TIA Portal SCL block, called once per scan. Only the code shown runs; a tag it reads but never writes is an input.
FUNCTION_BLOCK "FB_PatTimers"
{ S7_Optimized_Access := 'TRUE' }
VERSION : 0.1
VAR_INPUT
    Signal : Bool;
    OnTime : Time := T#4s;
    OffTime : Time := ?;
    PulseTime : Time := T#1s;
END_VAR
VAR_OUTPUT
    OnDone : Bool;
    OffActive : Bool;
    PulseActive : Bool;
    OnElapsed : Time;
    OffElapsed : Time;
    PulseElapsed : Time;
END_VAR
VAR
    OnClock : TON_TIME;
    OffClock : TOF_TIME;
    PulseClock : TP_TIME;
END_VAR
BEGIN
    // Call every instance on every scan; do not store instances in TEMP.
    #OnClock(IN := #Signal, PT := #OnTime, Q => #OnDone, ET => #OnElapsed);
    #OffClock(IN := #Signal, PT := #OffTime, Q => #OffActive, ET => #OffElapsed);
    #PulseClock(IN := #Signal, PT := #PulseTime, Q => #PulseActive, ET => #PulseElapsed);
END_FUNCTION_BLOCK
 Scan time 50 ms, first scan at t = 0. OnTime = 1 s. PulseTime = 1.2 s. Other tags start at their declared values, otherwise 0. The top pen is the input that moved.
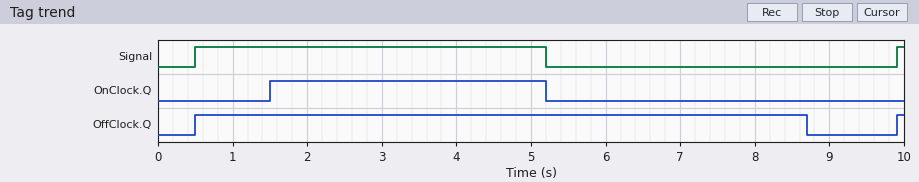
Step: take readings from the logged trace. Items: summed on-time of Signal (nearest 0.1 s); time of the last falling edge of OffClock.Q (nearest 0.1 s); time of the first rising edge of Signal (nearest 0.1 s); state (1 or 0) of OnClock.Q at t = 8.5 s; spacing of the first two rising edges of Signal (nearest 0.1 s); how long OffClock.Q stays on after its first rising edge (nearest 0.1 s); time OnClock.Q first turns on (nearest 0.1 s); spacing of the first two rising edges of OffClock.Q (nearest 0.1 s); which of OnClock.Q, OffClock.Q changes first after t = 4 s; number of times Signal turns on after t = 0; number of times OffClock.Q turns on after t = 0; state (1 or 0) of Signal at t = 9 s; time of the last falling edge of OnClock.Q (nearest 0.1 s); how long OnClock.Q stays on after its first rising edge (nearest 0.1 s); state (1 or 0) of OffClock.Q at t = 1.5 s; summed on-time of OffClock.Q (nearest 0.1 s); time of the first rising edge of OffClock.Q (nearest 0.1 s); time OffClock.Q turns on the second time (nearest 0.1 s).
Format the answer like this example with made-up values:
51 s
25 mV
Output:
4.8 s
8.7 s
0.5 s
0
9.4 s
8.2 s
1.5 s
9.4 s
OnClock.Q
2
2
0
5.2 s
3.7 s
1
8.3 s
0.5 s
9.9 s
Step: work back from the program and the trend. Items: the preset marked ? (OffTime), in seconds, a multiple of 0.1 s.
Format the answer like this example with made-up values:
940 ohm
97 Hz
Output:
3.5 s
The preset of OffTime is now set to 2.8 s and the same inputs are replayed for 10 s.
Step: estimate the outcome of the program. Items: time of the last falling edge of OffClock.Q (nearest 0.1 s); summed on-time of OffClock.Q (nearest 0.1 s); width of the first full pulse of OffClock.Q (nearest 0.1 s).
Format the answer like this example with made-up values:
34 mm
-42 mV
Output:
8.0 s
7.6 s
7.5 s
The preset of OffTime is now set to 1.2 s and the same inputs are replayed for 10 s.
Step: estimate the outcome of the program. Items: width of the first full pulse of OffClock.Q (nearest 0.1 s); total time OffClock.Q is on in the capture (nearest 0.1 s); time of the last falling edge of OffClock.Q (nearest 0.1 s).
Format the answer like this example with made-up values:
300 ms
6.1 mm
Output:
5.9 s
6.0 s
6.4 s
